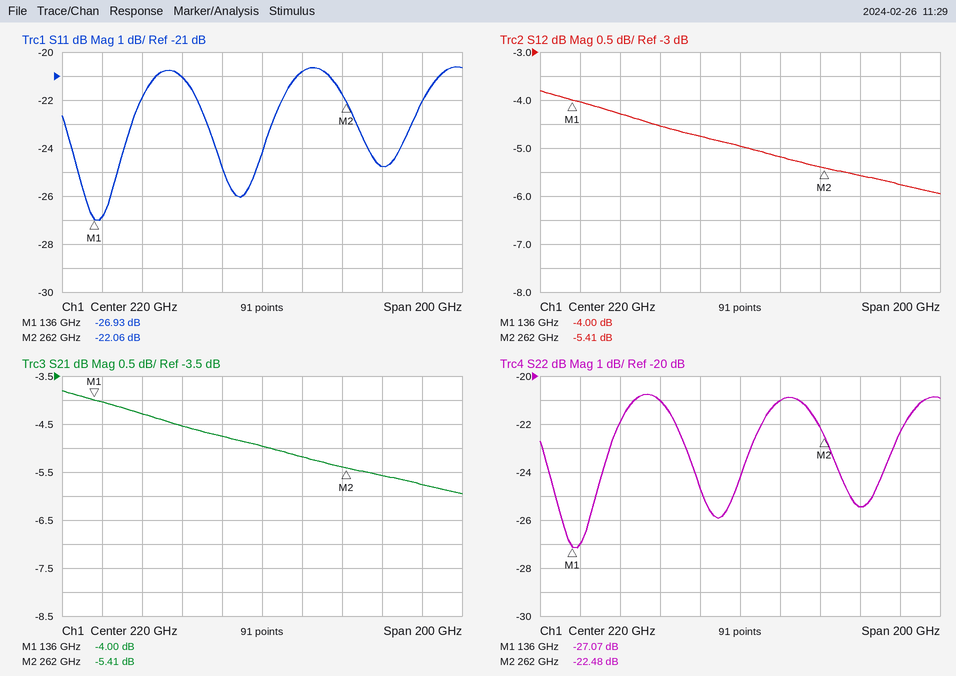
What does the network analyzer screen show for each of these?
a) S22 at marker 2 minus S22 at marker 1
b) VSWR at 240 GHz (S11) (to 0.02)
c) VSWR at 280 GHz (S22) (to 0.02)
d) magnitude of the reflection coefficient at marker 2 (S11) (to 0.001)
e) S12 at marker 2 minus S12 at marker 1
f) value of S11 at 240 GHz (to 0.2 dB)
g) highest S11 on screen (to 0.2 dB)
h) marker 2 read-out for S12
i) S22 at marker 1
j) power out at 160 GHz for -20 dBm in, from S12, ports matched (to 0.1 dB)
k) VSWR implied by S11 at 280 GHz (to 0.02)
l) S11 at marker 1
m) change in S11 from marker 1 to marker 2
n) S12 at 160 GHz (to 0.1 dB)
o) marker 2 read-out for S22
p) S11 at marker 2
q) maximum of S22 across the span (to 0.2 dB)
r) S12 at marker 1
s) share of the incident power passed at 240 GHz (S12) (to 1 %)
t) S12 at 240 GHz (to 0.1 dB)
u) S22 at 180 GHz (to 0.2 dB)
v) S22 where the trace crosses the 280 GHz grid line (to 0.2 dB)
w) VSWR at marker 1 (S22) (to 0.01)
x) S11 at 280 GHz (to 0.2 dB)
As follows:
4.59 dB
1.20
1.12
0.079
-1.41 dB
-20.8 dB
-20.6 dB
-5.41 dB
-27.07 dB
-24.3 dBm
1.12
-26.93 dB
4.87 dB
-4.3 dB
-22.48 dB
-22.06 dB
-20.8 dB
-4.00 dB
30 %
-5.2 dB
-21.0 dB
-25.4 dB
1.09
-24.8 dB
